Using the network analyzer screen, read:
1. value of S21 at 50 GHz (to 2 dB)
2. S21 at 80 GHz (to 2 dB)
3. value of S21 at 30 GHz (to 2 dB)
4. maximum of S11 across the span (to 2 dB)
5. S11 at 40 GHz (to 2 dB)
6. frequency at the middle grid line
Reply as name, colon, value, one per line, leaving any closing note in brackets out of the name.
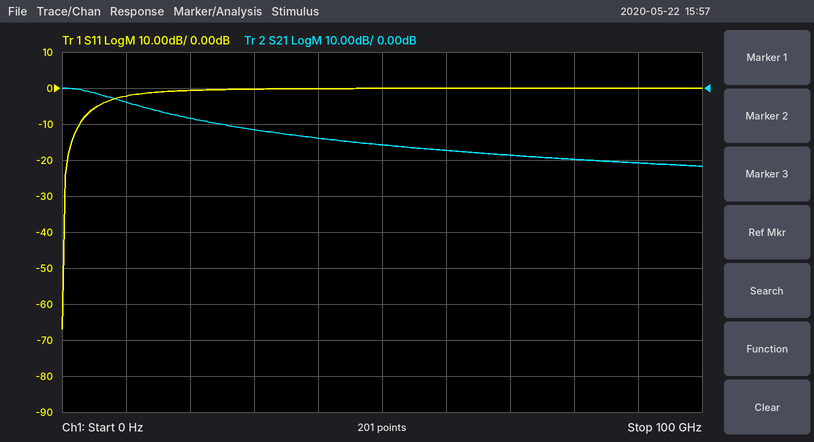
value of S21 at 50 GHz: -16 dB
S21 at 80 GHz: -20 dB
value of S21 at 30 GHz: -12 dB
maximum of S11 across the span: 0 dB
S11 at 40 GHz: 0 dB
frequency at the middle grid line: 50 GHz
